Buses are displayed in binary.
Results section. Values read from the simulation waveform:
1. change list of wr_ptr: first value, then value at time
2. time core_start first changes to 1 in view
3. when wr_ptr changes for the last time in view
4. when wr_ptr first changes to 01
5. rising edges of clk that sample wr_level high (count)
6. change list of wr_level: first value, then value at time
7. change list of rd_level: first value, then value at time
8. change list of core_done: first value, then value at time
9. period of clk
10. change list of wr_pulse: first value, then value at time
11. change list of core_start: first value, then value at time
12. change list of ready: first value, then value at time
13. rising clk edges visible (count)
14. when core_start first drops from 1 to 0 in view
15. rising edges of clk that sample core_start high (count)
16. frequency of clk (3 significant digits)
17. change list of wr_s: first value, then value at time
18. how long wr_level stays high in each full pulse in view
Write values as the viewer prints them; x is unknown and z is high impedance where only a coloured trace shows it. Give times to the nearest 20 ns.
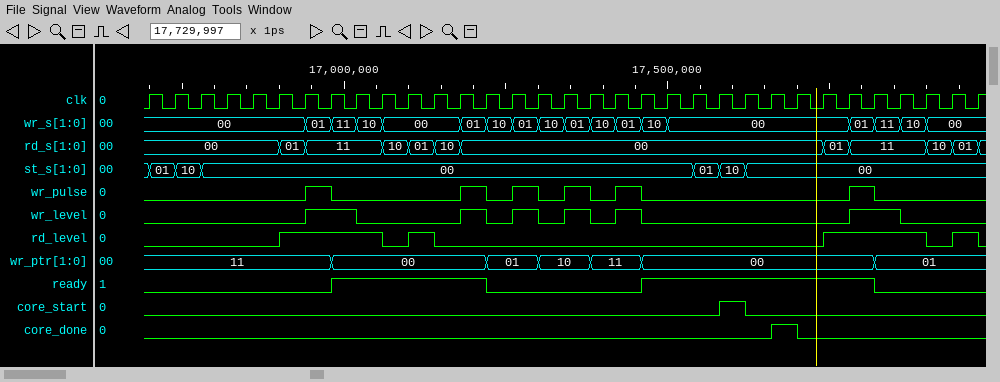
11, 00 at 16980 ns, 01 at 17220 ns, 10 at 17300 ns, 11 at 17380 ns, 00 at 17460 ns, 01 at 17820 ns
17580 ns
17820 ns
17220 ns
8
0, 1 at 16940 ns, 0 at 17020 ns, 1 at 17180 ns, 0 at 17220 ns, 1 at 17260 ns, 0 at 17300 ns, 1 at 17340 ns, 0 at 17380 ns, 1 at 17420 ns, 0 at 17460 ns, 1 at 17780 ns, 0 at 17860 ns
0, 1 at 16900 ns, 0 at 17060 ns, 1 at 17100 ns, 0 at 17140 ns, 1 at 17740 ns, 0 at 17900 ns, 1 at 17940 ns, 0 at 17980 ns
0, 1 at 17660 ns, 0 at 17700 ns
40 ns
0, 1 at 16940 ns, 0 at 16980 ns, 1 at 17180 ns, 0 at 17220 ns, 1 at 17260 ns, 0 at 17300 ns, 1 at 17340 ns, 0 at 17380 ns, 1 at 17420 ns, 0 at 17460 ns, 1 at 17780 ns, 0 at 17820 ns
0, 1 at 17580 ns, 0 at 17620 ns
0, 1 at 16980 ns, 0 at 17220 ns, 1 at 17460 ns, 0 at 17820 ns
33
17620 ns
1
25.0 MHz
00, 01 at 16940 ns, 11 at 16980 ns, 10 at 17020 ns, 00 at 17060 ns, 01 at 17180 ns, 10 at 17220 ns, 01 at 17260 ns, 10 at 17300 ns, 01 at 17340 ns, 10 at 17380 ns, 01 at 17420 ns, 10 at 17460 ns, 00 at 17500 ns, 01 at 17780 ns, 11 at 17820 ns, 10 at 17860 ns, 00 at 17900 ns
80 ns, 40 ns, 40 ns, 40 ns, 40 ns, 80 ns
